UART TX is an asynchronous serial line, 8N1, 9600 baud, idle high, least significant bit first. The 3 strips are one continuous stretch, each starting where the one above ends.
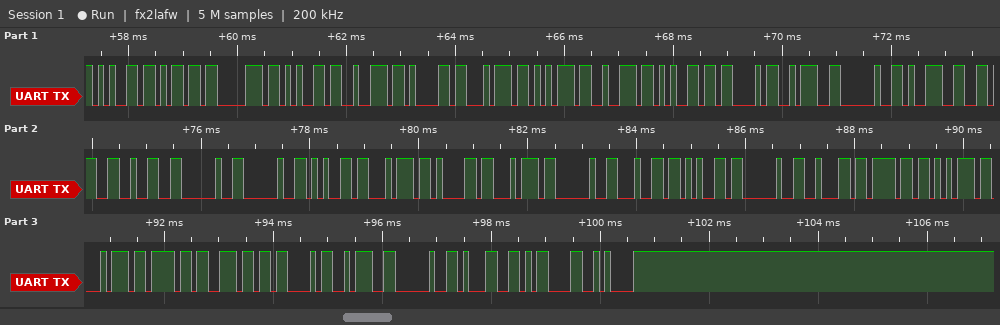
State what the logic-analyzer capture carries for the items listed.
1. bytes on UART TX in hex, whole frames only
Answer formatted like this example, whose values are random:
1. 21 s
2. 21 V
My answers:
1. 0x65 0x6D 0x70 0x65 0x72 0x61 0x74 0x75 0x72 0x65 0x43 0x3A 0x20 0x39 0x36 0x32 0x20 0x20 0x65 0x74 0x61 0x74 0x20 0x64 0x65 0x20 0x62 0x6F 0x75 0x74 0x6F 0x6E 0x43 0x3A 0x20 0x31 0x0D 0x0A
